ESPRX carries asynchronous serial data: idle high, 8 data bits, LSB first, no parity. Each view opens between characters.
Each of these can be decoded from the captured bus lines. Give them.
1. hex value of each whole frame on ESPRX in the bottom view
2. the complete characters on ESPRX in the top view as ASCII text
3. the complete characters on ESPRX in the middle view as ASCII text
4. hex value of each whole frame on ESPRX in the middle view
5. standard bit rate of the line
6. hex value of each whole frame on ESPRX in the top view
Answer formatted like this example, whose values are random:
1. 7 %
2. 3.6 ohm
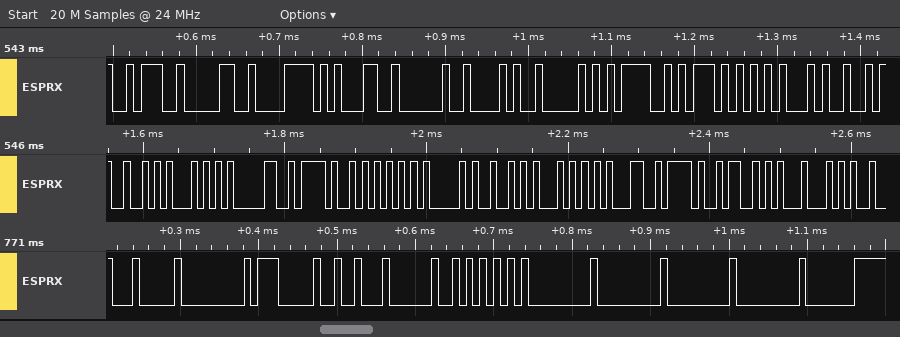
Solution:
1. 04, 00, 07, 12, 20, 55, 00, 00, 00, 00, C0
2. ":0x1 (POWE"
3. "RT0/UART1/SD"
4. 52, 54, 30, 2F, 55, 41, 52, 54, 31, 2F, 53, 44
5. 115200 baud
6. 3A, 30, 78, 31, 20, 28, 50, 4F, 57, 45
